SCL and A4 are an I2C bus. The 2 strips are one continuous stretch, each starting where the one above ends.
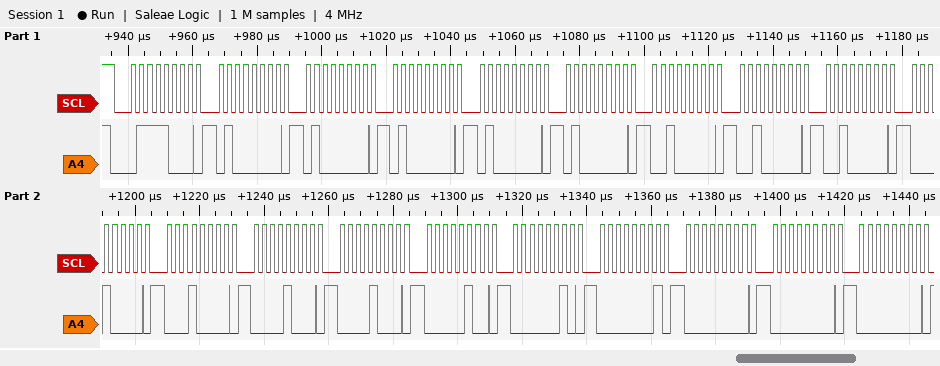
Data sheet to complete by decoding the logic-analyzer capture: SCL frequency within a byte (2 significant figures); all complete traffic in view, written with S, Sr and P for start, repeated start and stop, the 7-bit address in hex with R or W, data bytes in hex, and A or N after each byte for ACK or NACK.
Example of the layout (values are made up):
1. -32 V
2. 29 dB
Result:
1. 400 kHz
2. S 3CW A 40 A 40 A 40 A 40 A 40 A 20 A 20 A 20 A 10 A 10 A 08 A 08 A 04 A 02 A 01 A 00 A 00 A 00 A
